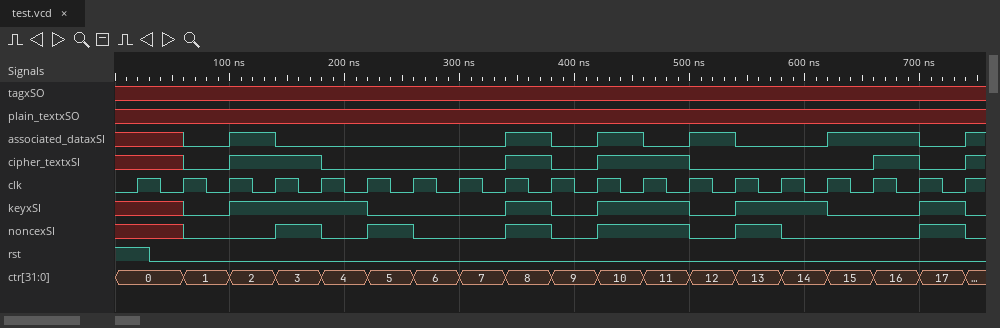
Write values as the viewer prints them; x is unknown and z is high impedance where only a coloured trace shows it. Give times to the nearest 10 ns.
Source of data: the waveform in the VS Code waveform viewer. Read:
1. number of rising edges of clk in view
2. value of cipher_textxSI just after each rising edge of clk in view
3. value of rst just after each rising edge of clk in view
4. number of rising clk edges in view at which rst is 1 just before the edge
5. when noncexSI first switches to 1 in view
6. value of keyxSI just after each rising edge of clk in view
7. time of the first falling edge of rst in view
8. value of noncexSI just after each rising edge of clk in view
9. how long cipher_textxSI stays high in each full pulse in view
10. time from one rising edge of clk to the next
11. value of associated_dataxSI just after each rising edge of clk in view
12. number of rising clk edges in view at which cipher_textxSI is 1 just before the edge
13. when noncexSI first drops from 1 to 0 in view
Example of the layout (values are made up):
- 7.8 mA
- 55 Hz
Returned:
- 19
- x 0 1 1 0 0 0 0 1 0 1 1 0 0 0 0 1 0 1
- 1 0 0 0 0 0 0 0 0 0 0 0 0 0 0 0 0 0 0
- 1
- 140 ns
- x 0 1 1 1 0 0 0 1 0 1 1 0 1 1 0 0 1 0
- 30 ns
- x 0 0 1 0 1 0 0 1 0 1 1 0 1 0 0 0 1 0
- 80 ns, 40 ns, 80 ns, 40 ns
- 40 ns
- x 0 1 0 0 0 0 0 1 0 1 0 1 0 0 1 1 0 1
- 6
- 180 ns
